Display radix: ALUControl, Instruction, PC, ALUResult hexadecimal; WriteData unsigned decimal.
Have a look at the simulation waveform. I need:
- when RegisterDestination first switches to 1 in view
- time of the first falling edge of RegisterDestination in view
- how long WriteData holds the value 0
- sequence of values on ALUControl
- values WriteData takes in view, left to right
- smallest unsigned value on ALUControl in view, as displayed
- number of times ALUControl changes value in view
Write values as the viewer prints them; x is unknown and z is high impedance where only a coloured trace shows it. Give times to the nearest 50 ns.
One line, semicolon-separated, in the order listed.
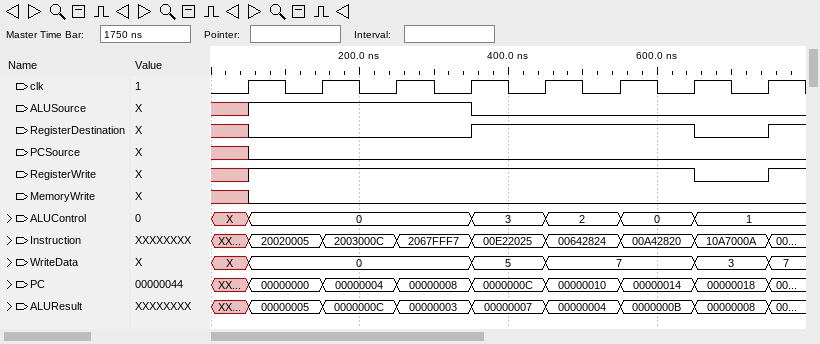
350 ns; 650 ns; 300 ns; X, 0, 3, 2, 0, 1; X, 0, 5, 7, 3, 7; 0; 5
